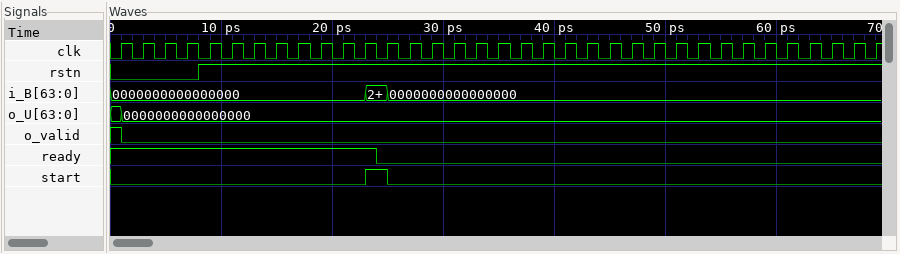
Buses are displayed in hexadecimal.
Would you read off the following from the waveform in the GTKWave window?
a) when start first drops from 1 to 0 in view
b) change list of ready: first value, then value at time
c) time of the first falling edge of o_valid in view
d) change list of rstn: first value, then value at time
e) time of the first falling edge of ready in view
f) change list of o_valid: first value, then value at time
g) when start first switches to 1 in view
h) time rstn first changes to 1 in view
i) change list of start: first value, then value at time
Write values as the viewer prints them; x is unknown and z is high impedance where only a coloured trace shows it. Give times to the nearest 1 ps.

25 ps
1, 0 at 24 ps
1 ps
0, 1 at 8 ps
24 ps
1, 0 at 1 ps
23 ps
8 ps
0, 1 at 23 ps, 0 at 25 ps
